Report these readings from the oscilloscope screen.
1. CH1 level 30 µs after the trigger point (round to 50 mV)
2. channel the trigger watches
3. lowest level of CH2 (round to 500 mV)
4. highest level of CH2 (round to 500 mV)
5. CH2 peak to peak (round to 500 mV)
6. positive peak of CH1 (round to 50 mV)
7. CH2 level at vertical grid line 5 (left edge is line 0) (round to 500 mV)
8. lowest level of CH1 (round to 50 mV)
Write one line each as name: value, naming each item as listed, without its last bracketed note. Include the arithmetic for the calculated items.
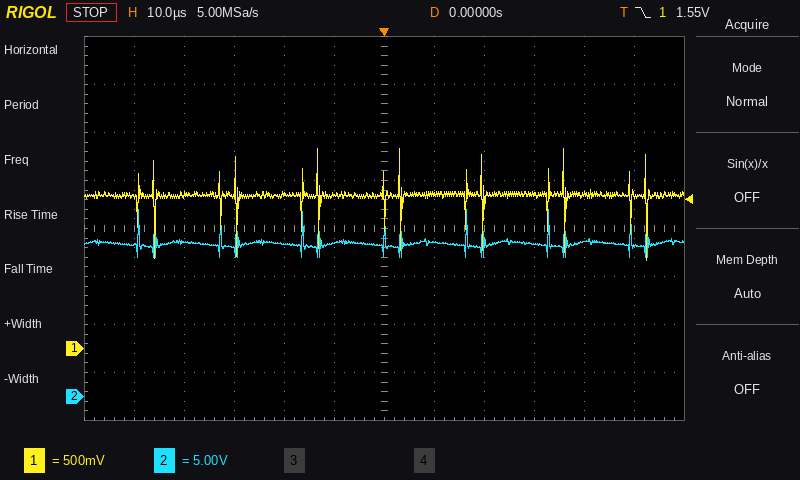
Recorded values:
CH1 level 30 µs after the trigger point: 1.60 V
channel the trigger watches: CH1
lowest level of CH2: 14.5 V
highest level of CH2: 19.5 V
CH2 peak to peak: 19.5 V − (14.5 V) = 5.0 V
positive peak of CH1: 2.10 V
CH2 level at vertical grid line 5 (left edge is line 0): 16.0 V
lowest level of CH1: 900 mV
